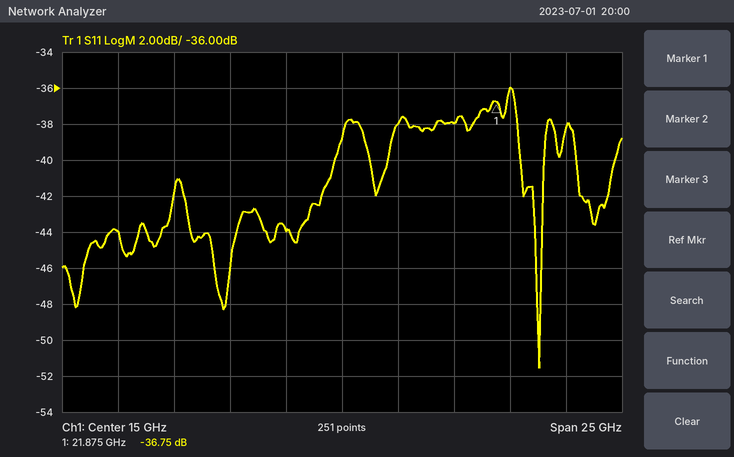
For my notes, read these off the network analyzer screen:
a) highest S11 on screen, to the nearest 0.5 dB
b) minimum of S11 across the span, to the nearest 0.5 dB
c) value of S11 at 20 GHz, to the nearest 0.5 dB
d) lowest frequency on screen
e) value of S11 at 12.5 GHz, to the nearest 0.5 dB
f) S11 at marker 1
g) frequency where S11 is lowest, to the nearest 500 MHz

-36.0 dB
-51.5 dB
-38.0 dB
2.5 GHz
-44.0 dB
-36.75 dB
24.0 GHz
